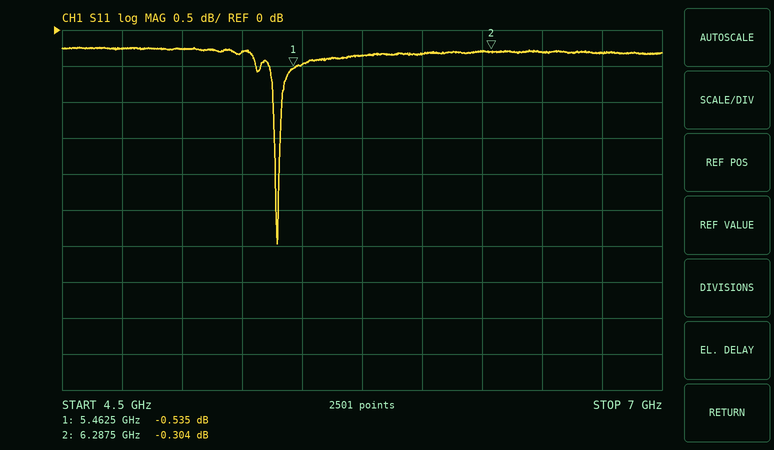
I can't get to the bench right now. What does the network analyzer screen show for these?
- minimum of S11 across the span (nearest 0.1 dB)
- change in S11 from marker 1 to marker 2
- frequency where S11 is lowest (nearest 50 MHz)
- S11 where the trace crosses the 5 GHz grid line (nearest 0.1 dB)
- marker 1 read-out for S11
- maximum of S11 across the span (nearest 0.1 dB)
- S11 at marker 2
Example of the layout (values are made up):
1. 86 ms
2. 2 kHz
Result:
1. -3.0 dB
2. 0.231 dB
3. 5.40 GHz
4. -0.3 dB
5. -0.535 dB
6. -0.2 dB
7. -0.304 dB
